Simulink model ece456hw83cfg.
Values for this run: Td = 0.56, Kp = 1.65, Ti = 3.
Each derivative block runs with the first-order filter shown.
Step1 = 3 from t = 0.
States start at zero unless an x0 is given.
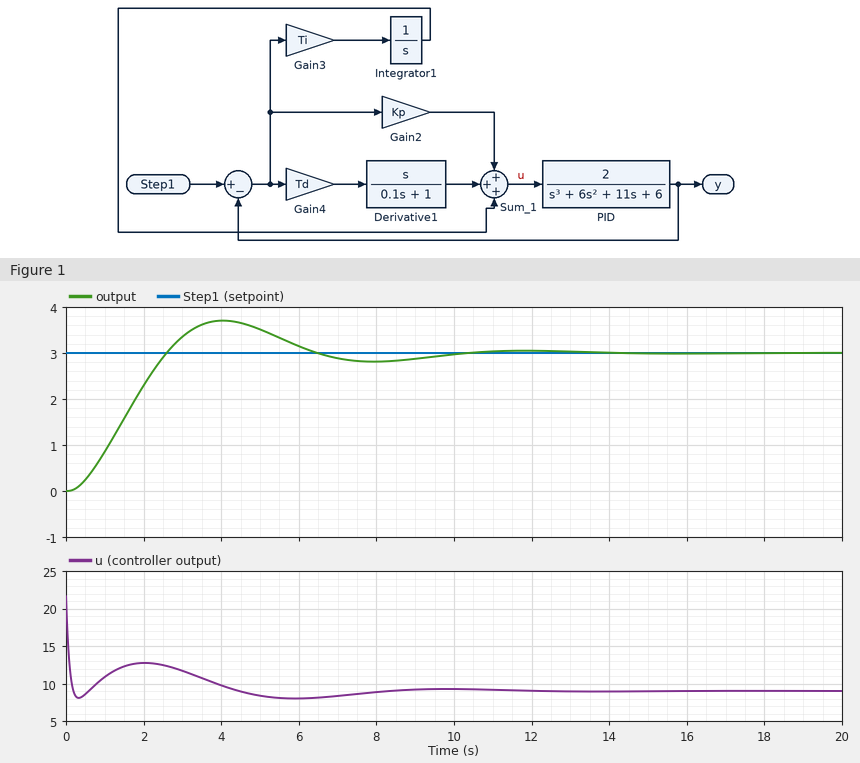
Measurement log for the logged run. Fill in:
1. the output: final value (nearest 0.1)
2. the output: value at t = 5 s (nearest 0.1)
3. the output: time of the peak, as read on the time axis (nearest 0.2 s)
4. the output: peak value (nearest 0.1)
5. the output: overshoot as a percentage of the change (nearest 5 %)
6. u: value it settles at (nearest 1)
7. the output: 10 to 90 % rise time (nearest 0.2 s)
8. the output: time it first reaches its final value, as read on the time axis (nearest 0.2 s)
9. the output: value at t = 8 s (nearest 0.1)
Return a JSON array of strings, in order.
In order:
["3.0", "3.5", "4.0 s", "3.7", "25 %", "9", "1.8 s", "2.6 s", "2.8"]
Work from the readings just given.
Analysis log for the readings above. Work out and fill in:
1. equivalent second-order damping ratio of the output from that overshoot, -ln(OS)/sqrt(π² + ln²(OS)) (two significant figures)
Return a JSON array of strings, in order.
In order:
["0.40"]
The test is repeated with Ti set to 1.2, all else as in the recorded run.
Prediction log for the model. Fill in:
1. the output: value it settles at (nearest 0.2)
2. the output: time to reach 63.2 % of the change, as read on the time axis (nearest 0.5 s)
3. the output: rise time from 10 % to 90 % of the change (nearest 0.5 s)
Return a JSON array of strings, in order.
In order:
["3.0", "2.5 s", "4.5 s"]
